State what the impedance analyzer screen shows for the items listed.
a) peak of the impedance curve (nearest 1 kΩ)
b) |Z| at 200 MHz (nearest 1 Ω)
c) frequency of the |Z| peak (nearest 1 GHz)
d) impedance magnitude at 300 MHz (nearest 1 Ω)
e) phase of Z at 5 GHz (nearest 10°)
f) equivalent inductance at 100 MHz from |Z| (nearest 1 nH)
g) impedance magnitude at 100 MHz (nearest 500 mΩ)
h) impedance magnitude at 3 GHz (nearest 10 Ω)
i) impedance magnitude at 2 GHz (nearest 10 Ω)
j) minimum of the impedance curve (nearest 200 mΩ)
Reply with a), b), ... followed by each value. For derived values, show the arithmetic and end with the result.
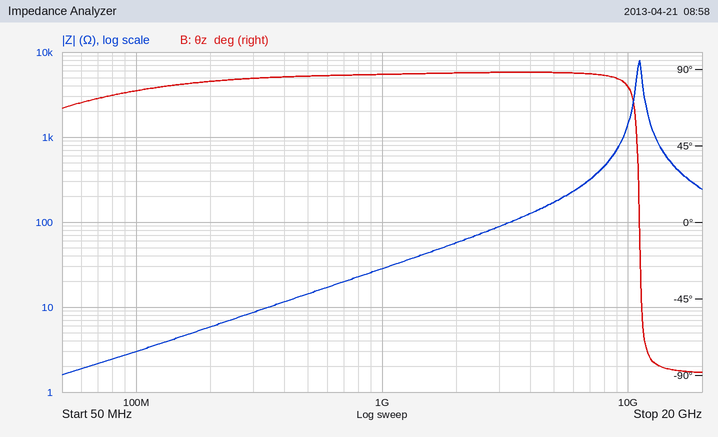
a) 8 kΩ
b) 6 Ω
c) 11 GHz
d) 9 Ω
e) 90°
f) L = 3.0 Ω/(2π × 100 MHz) ≈ 5 nH
g) 3.0 Ω
h) 90 Ω
i) 60 Ω
j) 1.6 Ω
